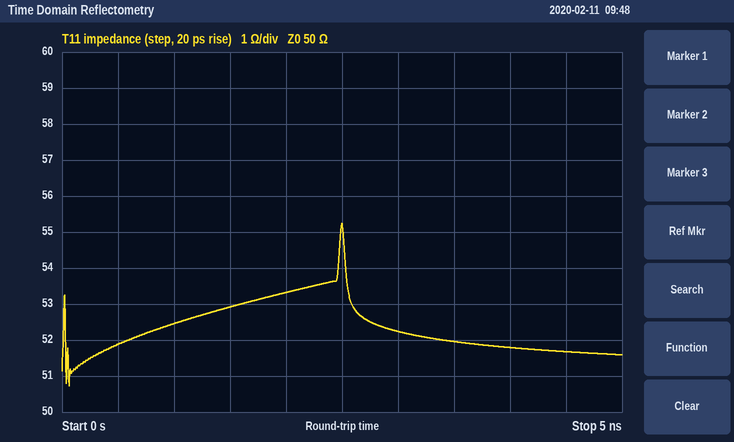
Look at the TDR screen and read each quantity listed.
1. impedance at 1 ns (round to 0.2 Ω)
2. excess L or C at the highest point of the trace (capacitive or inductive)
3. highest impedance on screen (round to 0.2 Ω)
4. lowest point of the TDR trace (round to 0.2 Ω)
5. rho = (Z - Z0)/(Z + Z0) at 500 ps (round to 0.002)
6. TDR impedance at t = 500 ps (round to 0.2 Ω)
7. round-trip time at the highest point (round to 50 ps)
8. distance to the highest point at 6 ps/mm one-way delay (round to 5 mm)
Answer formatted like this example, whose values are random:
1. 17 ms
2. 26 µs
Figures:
1. 52.4 Ω
2. inductive
3. 55.2 Ω
4. 50.8 Ω
5. +0.018
6. 51.8 Ω
7. 2.50 ns
8. 210 mm
